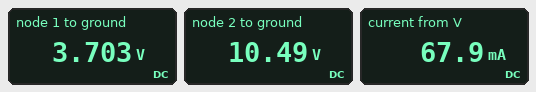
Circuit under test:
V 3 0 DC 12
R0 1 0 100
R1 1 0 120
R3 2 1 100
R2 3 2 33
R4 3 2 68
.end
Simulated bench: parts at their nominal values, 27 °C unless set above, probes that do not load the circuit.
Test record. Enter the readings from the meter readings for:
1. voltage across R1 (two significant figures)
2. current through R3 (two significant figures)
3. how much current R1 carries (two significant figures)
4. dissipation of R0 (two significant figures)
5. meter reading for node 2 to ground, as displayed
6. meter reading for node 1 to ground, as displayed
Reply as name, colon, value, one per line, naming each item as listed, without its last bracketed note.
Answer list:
voltage across R1: 3.7 V
current through R3: 68 mA
how much current R1 carries: 31 mA
dissipation of R0: 140 mW
meter reading for node 2 to ground, as displayed: 10.49 V
meter reading for node 1 to ground, as displayed: 3.703 V
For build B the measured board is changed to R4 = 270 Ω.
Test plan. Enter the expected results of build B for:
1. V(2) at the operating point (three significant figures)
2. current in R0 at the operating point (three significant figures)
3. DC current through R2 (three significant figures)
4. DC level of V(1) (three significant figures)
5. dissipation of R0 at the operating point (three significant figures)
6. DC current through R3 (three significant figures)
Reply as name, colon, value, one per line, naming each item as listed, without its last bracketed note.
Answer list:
V(2) at the operating point: 10.1 V
current in R0 at the operating point: 35.6 mA
DC current through R2: 58.1 mA
DC level of V(1): 3.56 V
dissipation of R0 at the operating point: 127 mW
DC current through R3: 65.2 mA
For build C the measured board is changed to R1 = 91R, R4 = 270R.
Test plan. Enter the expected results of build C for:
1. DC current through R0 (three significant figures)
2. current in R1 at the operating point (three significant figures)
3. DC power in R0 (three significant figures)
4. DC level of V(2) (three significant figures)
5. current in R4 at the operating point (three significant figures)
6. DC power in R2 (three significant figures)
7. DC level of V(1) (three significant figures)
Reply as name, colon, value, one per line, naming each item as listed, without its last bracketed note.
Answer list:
DC current through R0: 32.3 mA
current in R1 at the operating point: 35.5 mA
DC power in R0: 104 mW
DC level of V(2): 10.0 V
current in R4 at the operating point: 7.38 mA
DC power in R2: 120 mW
DC level of V(1): 3.23 V
